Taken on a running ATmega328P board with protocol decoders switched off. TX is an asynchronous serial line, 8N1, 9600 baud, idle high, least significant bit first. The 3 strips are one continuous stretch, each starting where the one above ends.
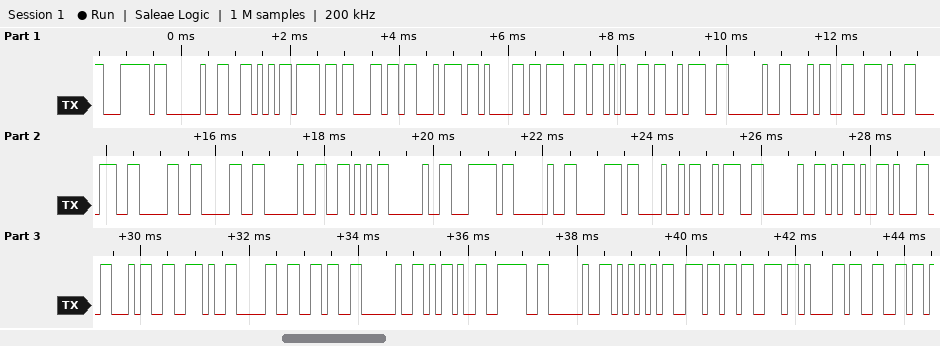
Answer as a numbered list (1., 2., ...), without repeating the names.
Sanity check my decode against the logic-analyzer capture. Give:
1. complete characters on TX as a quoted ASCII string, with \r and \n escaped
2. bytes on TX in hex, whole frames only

1. "| Voltage: 4.800 V | pH: -14.06 -> Unsaf"
2. 7C 20 56 6F 6C 74 61 67 65 3A 20 34 2E 38 30 30 20 56 20 7C 20 70 48 3A 20 2D 31 34 2E 30 36 20 2D 3E 20 55 6E 73 61 66
